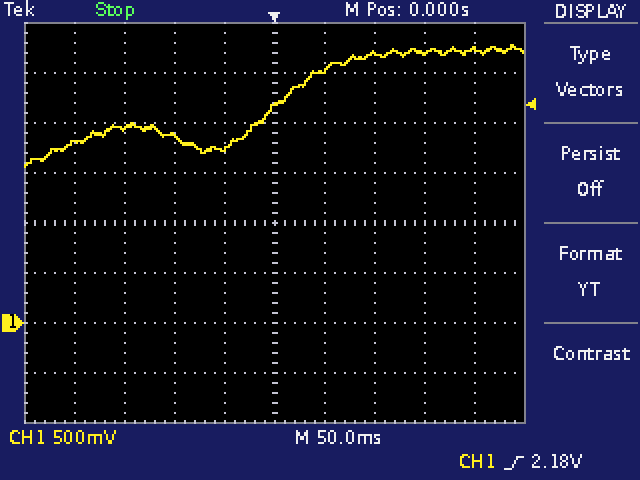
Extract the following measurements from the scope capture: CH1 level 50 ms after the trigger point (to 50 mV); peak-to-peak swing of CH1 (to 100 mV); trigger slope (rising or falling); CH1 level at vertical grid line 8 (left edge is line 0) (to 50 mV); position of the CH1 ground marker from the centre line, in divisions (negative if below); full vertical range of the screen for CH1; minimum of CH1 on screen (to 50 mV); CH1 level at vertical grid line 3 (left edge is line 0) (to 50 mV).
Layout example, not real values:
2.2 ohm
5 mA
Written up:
2.55 V
1.20 V
rising
2.70 V
-2.0 div
4 V
1.55 V
1.85 V
